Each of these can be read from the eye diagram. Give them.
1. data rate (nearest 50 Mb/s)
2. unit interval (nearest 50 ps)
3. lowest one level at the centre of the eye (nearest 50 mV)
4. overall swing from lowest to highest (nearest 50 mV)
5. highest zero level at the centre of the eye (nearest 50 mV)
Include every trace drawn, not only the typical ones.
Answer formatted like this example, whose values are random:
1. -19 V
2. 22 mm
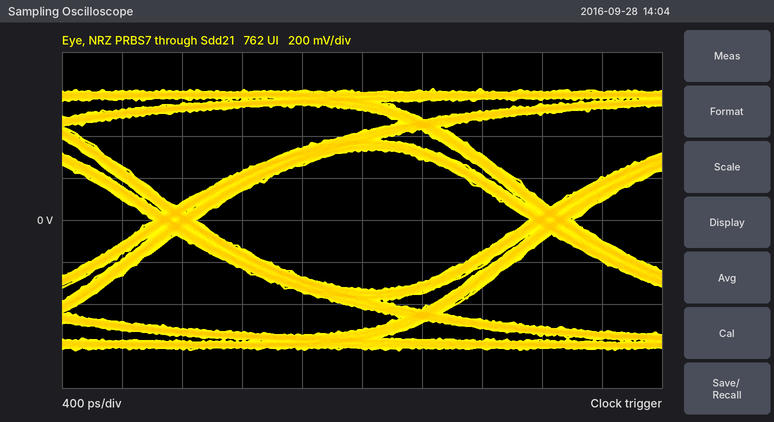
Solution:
1. 400 Mb/s
2. 2.50 ns
3. 350 mV
4. 1.25 V
5. -350 mV
